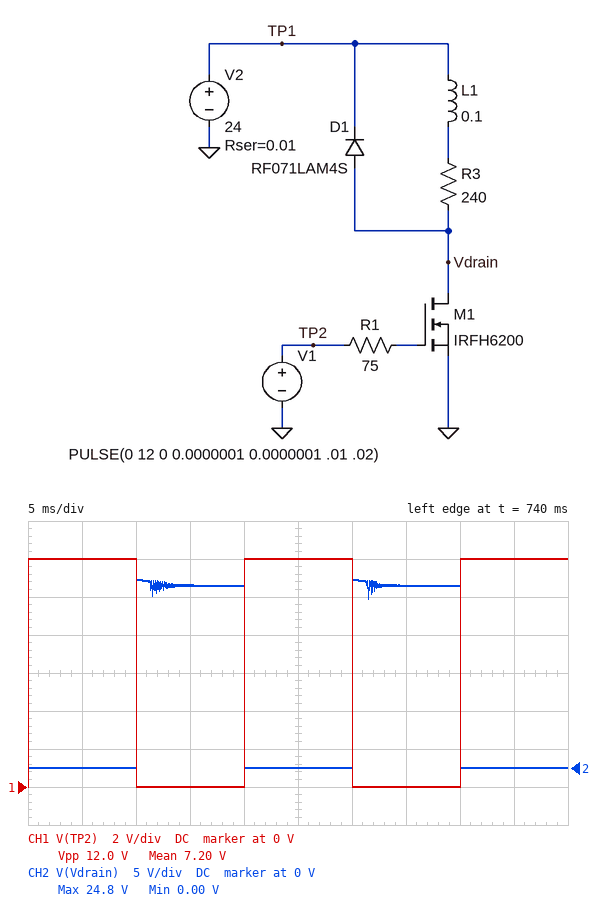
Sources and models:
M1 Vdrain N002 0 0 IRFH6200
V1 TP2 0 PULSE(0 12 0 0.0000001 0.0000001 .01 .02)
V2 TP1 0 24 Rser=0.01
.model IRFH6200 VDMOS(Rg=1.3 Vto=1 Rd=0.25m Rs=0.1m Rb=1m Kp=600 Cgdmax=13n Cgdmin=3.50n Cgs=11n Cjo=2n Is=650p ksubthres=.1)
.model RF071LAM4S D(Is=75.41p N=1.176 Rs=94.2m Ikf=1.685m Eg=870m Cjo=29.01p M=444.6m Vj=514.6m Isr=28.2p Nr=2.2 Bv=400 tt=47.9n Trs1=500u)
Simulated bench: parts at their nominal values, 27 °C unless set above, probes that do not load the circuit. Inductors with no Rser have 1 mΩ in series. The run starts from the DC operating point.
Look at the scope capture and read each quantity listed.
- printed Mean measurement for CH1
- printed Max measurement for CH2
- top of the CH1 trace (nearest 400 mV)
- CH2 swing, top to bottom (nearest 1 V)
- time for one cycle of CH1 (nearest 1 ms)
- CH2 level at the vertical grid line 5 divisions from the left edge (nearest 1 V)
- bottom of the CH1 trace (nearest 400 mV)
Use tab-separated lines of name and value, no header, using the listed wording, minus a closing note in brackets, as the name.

printed Mean measurement for CH1	7.20 V
printed Max measurement for CH2	24.8 V
top of the CH1 trace	12.0 V
CH2 swing, top to bottom	25 V
time for one cycle of CH1	20 ms
CH2 level at the vertical grid line 5 divisions from the left edge	0 V
bottom of the CH1 trace	0 V
